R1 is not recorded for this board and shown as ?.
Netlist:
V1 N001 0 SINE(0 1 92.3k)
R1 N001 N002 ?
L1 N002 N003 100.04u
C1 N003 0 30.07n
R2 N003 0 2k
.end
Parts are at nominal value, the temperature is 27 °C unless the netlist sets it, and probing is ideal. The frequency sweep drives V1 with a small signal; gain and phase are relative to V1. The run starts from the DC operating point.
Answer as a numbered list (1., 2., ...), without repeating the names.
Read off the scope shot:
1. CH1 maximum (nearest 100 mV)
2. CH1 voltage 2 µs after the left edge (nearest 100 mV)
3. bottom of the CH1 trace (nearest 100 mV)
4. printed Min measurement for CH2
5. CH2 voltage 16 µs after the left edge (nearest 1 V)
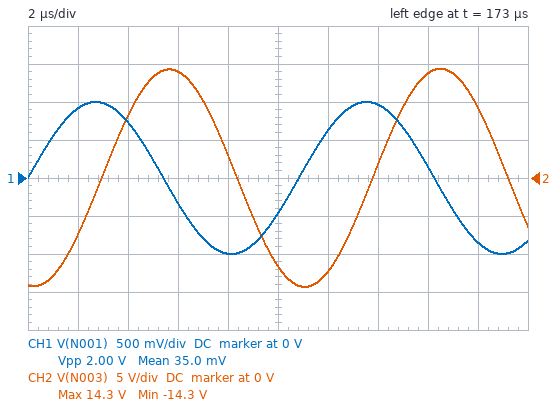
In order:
1. 1.0 V
2. 900 mV
3. -1.0 V
4. -14.3 V
5. 14 V
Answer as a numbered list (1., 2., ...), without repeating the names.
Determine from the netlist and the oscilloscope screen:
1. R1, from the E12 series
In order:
1. 2.2 Ω
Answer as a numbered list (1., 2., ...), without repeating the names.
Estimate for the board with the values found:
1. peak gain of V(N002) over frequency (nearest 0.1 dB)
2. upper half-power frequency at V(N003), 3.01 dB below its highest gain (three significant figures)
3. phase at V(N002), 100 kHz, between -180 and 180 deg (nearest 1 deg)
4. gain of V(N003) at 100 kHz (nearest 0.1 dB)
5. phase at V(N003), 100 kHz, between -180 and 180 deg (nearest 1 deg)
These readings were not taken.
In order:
1. 0 dB
2. 94.7 kHz
3. 12 deg
4. 14.0 dB
5. -159 deg
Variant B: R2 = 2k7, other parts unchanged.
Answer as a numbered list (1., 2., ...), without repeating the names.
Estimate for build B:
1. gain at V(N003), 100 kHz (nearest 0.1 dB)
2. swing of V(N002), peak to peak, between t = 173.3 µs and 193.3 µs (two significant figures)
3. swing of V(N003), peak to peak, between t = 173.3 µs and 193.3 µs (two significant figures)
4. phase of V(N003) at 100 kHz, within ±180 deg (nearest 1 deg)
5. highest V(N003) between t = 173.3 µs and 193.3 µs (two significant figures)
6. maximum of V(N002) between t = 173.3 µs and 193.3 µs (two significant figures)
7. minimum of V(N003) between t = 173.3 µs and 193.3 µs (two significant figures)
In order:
1. 14.1 dB
2. 830 mV
3. 32 V
4. -161 deg
5. 16 V
6. 420 mV
7. -16 V
